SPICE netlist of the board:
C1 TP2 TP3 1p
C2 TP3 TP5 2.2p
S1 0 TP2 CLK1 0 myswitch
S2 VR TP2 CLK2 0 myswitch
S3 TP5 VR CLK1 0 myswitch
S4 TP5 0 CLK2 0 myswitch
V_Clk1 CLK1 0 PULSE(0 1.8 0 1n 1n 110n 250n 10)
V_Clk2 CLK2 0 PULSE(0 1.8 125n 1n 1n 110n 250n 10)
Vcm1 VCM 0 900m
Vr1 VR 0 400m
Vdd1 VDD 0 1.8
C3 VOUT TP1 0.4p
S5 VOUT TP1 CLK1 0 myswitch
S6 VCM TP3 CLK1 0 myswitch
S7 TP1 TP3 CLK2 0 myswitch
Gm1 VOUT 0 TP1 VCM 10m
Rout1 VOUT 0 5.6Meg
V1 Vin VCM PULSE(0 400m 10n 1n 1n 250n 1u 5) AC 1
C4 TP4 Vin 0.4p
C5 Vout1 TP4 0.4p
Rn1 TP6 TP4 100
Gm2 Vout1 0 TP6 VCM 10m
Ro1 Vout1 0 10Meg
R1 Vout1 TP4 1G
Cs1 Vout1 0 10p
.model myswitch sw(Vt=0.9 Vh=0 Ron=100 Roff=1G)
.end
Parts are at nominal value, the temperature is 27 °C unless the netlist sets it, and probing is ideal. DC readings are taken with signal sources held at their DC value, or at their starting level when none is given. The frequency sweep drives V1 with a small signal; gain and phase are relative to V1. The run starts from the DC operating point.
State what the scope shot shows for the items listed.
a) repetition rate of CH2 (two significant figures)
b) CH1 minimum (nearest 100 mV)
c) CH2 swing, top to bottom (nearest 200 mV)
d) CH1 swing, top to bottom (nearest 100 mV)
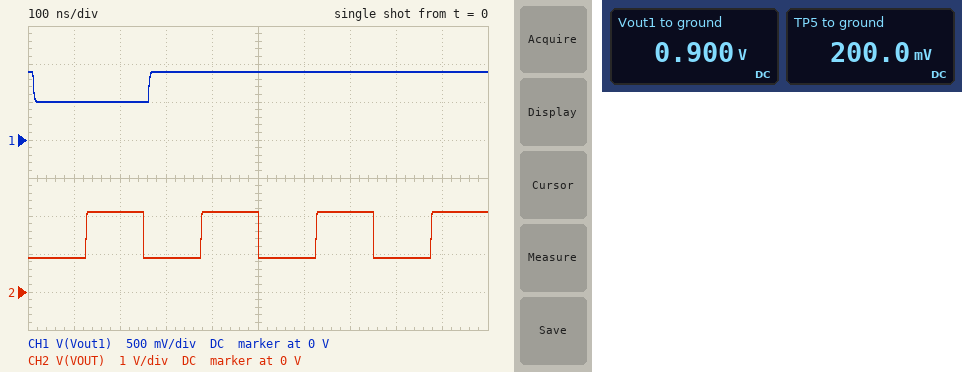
4.0 MHz
500 mV
1.2 V
400 mV
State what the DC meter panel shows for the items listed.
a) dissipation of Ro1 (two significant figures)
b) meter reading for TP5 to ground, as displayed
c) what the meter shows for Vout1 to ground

81 nW
200.0 mV
0.900 V
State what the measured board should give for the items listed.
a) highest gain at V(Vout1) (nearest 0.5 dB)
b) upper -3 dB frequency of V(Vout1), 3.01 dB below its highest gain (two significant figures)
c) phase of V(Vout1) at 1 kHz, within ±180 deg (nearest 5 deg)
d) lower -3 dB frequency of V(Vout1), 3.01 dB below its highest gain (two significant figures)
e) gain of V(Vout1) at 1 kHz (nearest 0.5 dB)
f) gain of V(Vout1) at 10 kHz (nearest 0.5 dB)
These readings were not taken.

0 dB
78 MHz
-160 deg
400 Hz
-0.5 dB
0 dB
